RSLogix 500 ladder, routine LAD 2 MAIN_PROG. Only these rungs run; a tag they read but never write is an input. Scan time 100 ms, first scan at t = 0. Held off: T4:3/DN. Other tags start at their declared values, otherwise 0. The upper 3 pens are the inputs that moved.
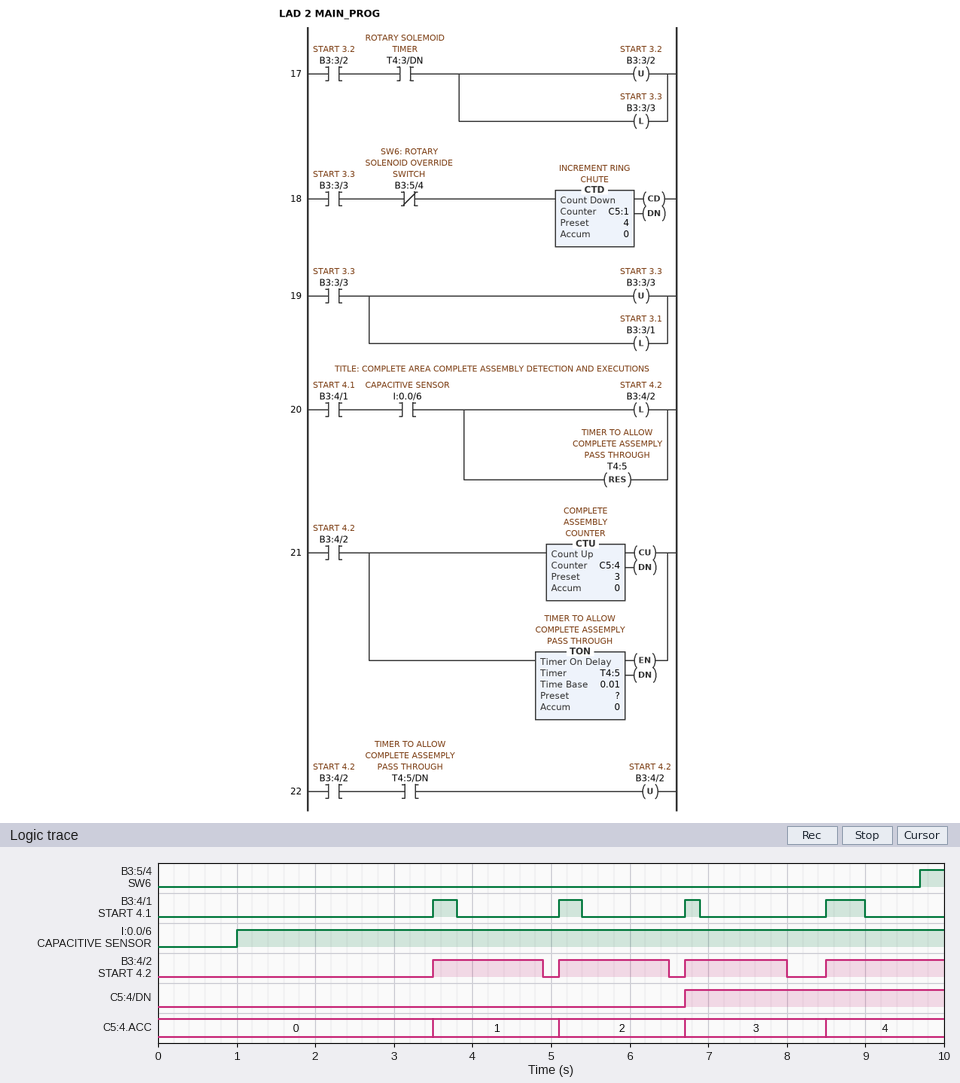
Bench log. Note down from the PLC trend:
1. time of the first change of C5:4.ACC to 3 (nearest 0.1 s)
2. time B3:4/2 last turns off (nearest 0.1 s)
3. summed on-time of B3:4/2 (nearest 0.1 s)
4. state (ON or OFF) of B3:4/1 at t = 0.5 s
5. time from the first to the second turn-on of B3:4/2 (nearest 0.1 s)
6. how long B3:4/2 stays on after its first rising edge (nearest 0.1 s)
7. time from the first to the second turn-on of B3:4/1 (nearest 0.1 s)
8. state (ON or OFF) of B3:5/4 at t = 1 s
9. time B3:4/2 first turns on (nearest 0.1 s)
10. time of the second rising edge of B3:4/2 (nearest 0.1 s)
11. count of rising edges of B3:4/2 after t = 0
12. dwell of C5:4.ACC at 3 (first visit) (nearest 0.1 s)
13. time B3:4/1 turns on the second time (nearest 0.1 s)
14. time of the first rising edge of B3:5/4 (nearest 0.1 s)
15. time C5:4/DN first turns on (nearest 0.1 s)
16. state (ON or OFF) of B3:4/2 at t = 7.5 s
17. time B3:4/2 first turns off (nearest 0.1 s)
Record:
6.7 s
8.0 s
5.6 s
OFF
1.6 s
1.4 s
1.6 s
OFF
3.5 s
5.1 s
4
1.8 s
5.1 s
9.7 s
6.7 s
ON
4.9 s
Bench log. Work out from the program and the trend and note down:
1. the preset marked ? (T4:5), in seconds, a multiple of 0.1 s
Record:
1.2 s
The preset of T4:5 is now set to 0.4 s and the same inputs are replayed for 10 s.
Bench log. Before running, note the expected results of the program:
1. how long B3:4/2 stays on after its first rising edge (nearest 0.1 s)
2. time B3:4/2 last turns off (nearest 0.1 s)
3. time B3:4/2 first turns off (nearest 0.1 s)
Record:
0.6 s
9.3 s
4.1 s
